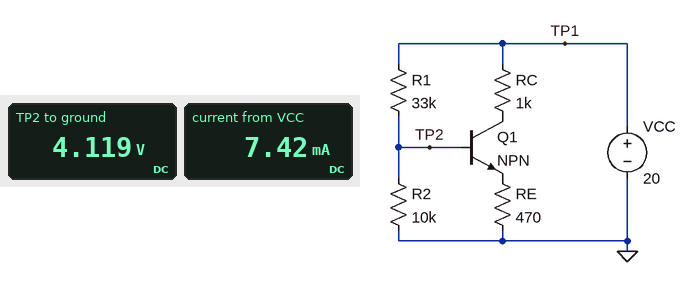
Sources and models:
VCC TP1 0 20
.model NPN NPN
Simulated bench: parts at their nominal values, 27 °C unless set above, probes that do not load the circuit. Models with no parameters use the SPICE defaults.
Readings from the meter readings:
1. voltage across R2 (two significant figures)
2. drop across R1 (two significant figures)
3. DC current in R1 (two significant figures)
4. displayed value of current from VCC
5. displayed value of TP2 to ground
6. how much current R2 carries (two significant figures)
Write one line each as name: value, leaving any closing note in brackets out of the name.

voltage across R2: 4.1 V
drop across R1: 16 V
DC current in R1: 480 µA
displayed value of current from VCC: 7.42 mA
displayed value of TP2 to ground: 4.119 V
how much current R2 carries: 410 µA
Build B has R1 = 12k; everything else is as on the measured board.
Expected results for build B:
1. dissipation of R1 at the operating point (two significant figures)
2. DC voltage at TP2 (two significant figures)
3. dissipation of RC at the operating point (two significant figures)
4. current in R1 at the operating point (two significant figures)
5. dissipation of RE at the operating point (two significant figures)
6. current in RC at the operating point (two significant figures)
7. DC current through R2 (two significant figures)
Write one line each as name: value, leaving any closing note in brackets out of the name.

dissipation of R1 at the operating point: 13 mW
DC voltage at TP2: 7.3 V
dissipation of RC at the operating point: 180 mW
current in R1 at the operating point: 1.1 mA
dissipation of RE at the operating point: 89 mW
current in RC at the operating point: 13 mA
DC current through R2: 730 µA
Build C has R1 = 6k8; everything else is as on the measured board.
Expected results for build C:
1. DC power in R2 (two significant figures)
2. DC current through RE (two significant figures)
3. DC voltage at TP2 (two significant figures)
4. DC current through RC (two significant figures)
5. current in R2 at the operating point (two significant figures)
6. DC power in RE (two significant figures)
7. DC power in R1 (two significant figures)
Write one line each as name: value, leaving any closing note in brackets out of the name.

DC power in R2: 5.7 mW
DC current through RE: 14 mA
DC voltage at TP2: 7.6 V
DC current through RC: 13 mA
current in R2 at the operating point: 760 µA
DC power in RE: 96 mW
DC power in R1: 23 mW
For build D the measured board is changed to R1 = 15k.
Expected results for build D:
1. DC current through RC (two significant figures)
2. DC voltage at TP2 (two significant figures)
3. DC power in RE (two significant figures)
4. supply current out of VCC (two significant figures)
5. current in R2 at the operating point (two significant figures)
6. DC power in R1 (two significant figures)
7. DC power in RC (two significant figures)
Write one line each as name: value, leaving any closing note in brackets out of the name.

DC current through RC: 13 mA
DC voltage at TP2: 7.2 V
DC power in RE: 86 mW
supply current out of VCC: 14 mA
current in R2 at the operating point: 720 µA
DC power in R1: 11 mW
DC power in RC: 180 mW
